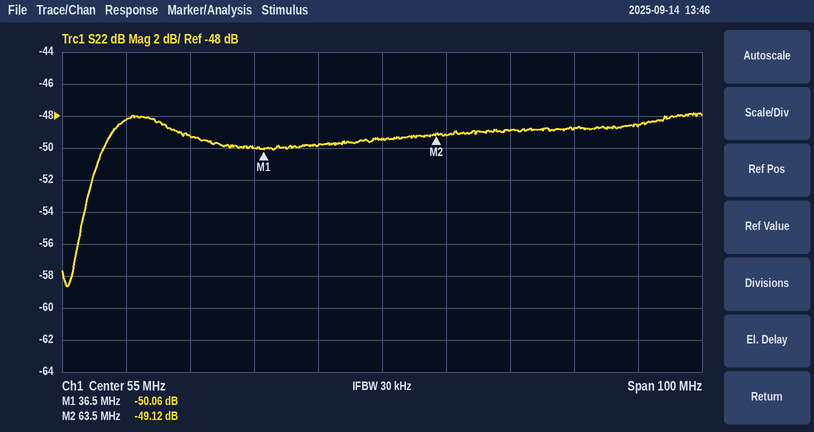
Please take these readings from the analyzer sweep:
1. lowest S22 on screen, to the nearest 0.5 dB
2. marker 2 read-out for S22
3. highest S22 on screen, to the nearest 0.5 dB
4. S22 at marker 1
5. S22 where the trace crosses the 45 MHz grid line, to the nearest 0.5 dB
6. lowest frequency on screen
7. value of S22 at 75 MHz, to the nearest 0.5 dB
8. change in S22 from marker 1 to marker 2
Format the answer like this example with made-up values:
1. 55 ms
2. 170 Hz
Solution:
1. -58.5 dB
2. -49.12 dB
3. -48.0 dB
4. -50.06 dB
5. -50.0 dB
6. 5 MHz
7. -49.0 dB
8. 0.94 dB
